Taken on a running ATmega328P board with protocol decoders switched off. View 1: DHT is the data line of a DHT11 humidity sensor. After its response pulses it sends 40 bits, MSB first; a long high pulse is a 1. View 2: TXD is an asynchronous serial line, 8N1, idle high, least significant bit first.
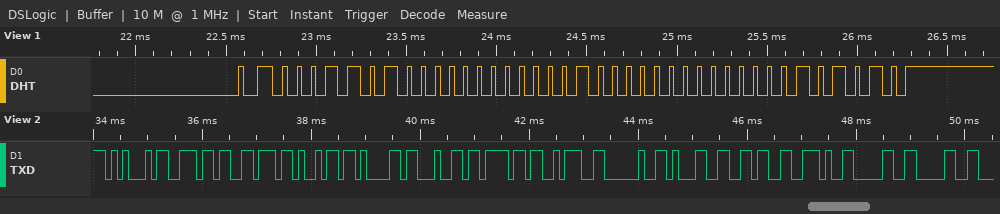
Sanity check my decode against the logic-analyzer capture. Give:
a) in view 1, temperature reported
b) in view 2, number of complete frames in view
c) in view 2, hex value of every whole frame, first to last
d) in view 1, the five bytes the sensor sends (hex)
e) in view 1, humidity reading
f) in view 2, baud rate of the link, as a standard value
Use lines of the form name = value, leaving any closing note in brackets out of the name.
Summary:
in view 1, temperature reported = 16.0 °C
in view 2, number of complete frames in view = 14
in view 2, hex value of every whole frame, first to last = 0x45 0x6E 0x76 0x69 0x61 0x64 0x6F 0x3A 0x20 0x31 0x36 0x2E 0x30 0x30
in view 1, the five bytes the sensor sends = 1A 00 10 00 2A
in view 1, humidity reading = 26 %
in view 2, baud rate of the link, as a standard value = 9600 baud
